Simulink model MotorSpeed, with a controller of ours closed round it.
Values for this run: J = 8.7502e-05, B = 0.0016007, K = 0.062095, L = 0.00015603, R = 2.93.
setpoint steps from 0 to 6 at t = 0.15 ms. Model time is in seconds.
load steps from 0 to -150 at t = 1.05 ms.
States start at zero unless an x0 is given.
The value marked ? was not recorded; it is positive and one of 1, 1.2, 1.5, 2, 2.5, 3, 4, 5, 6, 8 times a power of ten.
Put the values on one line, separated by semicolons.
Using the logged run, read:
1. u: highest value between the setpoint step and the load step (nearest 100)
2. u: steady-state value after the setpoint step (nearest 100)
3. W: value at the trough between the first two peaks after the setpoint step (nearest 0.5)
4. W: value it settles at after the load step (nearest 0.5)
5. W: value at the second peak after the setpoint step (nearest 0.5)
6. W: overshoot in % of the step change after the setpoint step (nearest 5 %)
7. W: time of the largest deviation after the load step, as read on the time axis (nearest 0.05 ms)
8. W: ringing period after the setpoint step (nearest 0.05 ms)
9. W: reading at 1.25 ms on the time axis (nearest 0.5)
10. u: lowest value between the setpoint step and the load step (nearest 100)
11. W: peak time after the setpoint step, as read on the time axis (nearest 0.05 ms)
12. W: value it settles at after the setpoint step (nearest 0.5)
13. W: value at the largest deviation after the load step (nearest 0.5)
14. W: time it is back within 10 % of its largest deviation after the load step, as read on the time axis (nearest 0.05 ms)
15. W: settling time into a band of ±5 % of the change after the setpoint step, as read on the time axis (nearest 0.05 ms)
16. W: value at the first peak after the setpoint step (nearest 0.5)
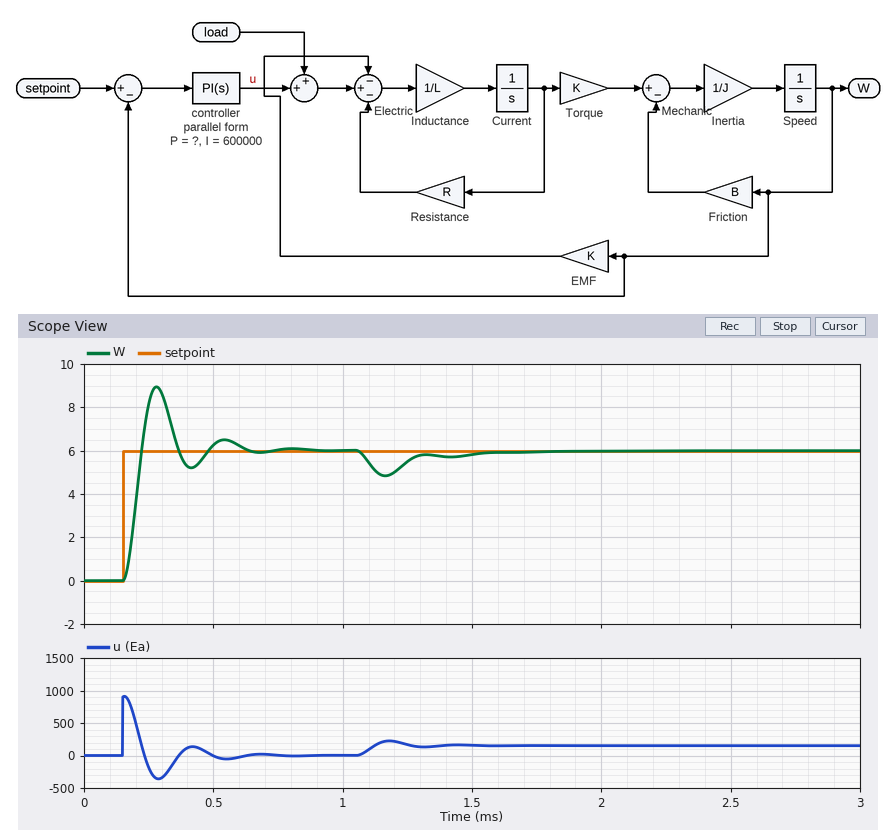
900; 0; 5.0; 6.0; 6.5; 50 %; 1.15 ms; 0.25 ms; 5.5; -400; 0.30 ms; 6.0; 5.0; 1.55 ms; 0.60 ms; 9.0
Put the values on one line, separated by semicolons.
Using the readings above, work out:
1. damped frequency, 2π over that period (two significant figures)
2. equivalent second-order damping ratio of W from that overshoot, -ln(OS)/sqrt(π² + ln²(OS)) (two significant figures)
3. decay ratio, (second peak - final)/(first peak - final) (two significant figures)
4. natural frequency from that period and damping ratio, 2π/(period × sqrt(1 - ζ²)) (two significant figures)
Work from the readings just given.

25 rad/ms; 0.22; 0.17; 26 rad/ms
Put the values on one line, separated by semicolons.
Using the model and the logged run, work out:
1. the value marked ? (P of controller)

150
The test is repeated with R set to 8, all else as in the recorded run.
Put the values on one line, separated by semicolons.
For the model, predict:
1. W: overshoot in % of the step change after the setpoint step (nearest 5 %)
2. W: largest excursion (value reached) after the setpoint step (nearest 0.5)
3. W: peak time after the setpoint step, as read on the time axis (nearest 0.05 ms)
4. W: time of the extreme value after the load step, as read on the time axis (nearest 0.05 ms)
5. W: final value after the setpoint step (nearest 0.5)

20 %; 7.0; 0.40 ms; 1.20 ms; 6.0
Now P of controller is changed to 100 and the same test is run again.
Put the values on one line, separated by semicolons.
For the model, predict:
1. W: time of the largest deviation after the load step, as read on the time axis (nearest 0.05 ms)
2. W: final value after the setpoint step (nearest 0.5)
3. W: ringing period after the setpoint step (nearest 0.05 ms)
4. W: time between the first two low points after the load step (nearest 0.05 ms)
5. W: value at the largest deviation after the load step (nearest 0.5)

1.20 ms; 6.0; 0.35 ms; 0.35 ms; 4.5
